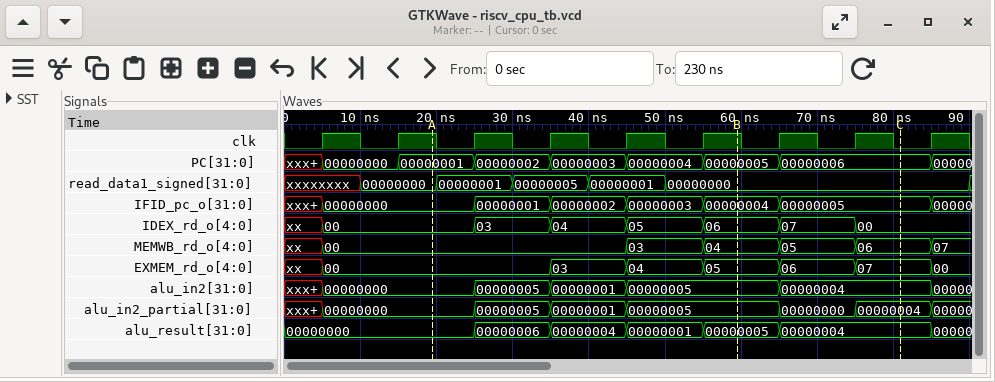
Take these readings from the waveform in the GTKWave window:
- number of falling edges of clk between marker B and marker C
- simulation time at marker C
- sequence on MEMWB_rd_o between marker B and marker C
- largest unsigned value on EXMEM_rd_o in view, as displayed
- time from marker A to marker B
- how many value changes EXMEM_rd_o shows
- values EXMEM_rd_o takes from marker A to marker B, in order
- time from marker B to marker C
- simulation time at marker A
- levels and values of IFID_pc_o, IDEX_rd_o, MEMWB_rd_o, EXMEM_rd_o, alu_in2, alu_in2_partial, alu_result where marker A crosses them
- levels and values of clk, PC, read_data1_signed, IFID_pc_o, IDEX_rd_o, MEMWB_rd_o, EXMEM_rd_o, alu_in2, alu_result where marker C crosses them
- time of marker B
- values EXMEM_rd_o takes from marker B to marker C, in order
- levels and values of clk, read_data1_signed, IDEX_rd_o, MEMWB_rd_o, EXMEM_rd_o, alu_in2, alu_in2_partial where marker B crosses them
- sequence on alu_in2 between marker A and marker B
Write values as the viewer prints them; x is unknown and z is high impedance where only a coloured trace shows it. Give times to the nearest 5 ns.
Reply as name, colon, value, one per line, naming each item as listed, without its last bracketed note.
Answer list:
number of falling edges of clk between marker B and marker C: 3
simulation time at marker C: 80 ns
sequence on MEMWB_rd_o between marker B and marker C: 04, 05, 06
largest unsigned value on EXMEM_rd_o in view, as displayed: 07
time from marker A to marker B: 40 ns
how many value changes EXMEM_rd_o shows: 7
values EXMEM_rd_o takes from marker A to marker B, in order: 00, 03, 04, 05
time from marker B to marker C: 20 ns
simulation time at marker A: 20 ns
levels and values of IFID_pc_o, IDEX_rd_o, MEMWB_rd_o, EXMEM_rd_o, alu_in2, alu_in2_partial, alu_result where marker A crosses them: IFID_pc_o=00000000, IDEX_rd_o=00, MEMWB_rd_o=00, EXMEM_rd_o=00, alu_in2=00000000, alu_in2_partial=00000000, alu_result=00000000
levels and values of clk, PC, read_data1_signed, IFID_pc_o, IDEX_rd_o, MEMWB_rd_o, EXMEM_rd_o, alu_in2, alu_result where marker C crosses them: clk=0, PC=00000006, read_data1_signed=00000000, IFID_pc_o=00000005, IDEX_rd_o=00, MEMWB_rd_o=06, EXMEM_rd_o=07, alu_in2=00000004, alu_result=00000004
time of marker B: 60 ns
values EXMEM_rd_o takes from marker B to marker C, in order: 05, 06, 07
levels and values of clk, read_data1_signed, IDEX_rd_o, MEMWB_rd_o, EXMEM_rd_o, alu_in2, alu_in2_partial where marker B crosses them: clk=1, read_data1_signed=00000000, IDEX_rd_o=06, MEMWB_rd_o=04, EXMEM_rd_o=05, alu_in2=00000005, alu_in2_partial=00000005
sequence on alu_in2 between marker A and marker B: 00000000, 00000005, 00000001, 00000005
